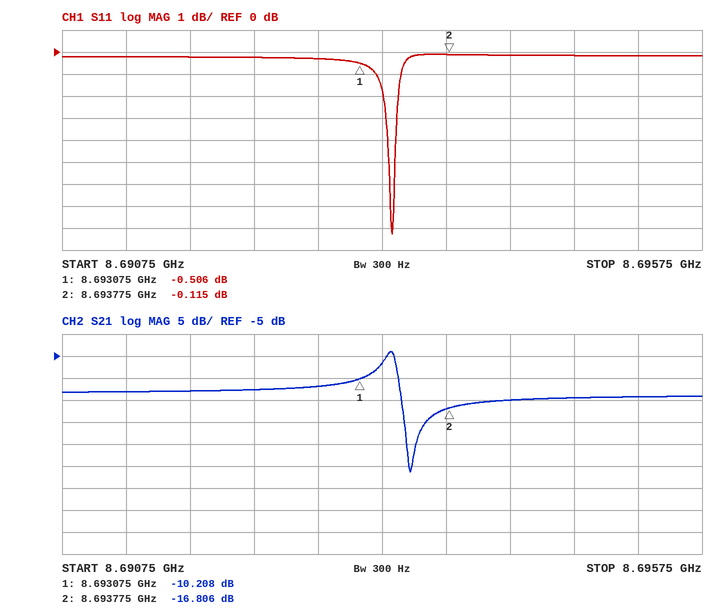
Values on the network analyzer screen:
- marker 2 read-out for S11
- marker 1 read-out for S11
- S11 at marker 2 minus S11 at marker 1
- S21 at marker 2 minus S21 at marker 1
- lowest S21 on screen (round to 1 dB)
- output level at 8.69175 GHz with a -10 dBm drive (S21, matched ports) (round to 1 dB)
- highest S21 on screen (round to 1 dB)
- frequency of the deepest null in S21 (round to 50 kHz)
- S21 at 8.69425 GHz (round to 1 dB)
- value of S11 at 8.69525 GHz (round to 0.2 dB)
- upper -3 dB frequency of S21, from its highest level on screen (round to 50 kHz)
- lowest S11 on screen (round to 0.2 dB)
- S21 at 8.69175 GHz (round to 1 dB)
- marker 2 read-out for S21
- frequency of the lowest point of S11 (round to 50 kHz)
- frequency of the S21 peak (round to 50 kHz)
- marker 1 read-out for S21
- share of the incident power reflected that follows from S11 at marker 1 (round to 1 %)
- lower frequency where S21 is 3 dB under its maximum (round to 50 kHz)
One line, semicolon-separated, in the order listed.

-0.115 dB; -0.506 dB; 0.391 dB; -6.598 dB; -31 dB; -23 dBm; -4 dB; 8.69345 GHz; -15 dB; -0.2 dB; 8.69335 GHz; -8.2 dB; -13 dB; -16.806 dB; 8.69335 GHz; 8.69330 GHz; -10.208 dB; 89 %; 8.69325 GHz
